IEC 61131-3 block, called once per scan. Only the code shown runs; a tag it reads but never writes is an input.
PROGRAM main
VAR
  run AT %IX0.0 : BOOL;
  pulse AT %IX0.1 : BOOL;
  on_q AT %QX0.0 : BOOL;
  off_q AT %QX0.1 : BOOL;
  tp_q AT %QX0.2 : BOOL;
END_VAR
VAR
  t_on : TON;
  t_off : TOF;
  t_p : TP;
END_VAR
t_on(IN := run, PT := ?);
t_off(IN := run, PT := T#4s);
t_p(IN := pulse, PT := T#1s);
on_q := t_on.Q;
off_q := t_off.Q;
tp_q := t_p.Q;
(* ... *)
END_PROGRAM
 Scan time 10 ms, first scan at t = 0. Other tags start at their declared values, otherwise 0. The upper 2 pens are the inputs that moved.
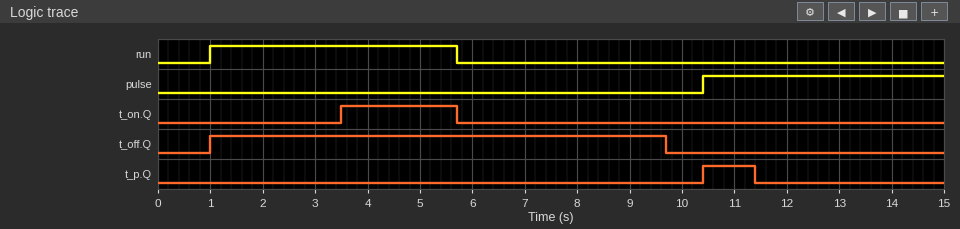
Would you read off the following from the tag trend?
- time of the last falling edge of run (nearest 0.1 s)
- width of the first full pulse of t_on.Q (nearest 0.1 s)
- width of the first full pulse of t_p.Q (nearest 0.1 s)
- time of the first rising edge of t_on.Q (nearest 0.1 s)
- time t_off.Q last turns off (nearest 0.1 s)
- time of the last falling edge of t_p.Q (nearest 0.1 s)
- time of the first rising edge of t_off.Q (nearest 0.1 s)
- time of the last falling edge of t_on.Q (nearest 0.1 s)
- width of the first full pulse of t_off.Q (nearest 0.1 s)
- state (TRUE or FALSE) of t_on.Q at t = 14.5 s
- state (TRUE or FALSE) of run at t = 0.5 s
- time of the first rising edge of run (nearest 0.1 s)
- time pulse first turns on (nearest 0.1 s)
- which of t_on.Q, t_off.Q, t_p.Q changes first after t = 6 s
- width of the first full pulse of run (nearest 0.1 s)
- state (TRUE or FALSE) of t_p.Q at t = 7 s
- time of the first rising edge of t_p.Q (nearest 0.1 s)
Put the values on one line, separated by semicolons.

5.7 s; 2.2 s; 1.0 s; 3.5 s; 9.7 s; 11.4 s; 1.0 s; 5.7 s; 8.7 s; FALSE; FALSE; 1.0 s; 10.4 s; t_off.Q; 4.7 s; FALSE; 10.4 s
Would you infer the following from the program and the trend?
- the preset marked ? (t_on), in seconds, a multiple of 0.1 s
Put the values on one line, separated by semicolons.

2.5 s
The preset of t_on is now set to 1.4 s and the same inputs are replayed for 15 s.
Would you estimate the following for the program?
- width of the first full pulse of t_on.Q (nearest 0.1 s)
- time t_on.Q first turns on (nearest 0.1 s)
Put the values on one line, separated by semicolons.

3.3 s; 2.4 s
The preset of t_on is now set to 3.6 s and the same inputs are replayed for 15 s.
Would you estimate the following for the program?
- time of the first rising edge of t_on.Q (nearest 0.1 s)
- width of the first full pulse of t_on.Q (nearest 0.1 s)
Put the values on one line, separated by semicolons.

4.6 s; 1.1 s
